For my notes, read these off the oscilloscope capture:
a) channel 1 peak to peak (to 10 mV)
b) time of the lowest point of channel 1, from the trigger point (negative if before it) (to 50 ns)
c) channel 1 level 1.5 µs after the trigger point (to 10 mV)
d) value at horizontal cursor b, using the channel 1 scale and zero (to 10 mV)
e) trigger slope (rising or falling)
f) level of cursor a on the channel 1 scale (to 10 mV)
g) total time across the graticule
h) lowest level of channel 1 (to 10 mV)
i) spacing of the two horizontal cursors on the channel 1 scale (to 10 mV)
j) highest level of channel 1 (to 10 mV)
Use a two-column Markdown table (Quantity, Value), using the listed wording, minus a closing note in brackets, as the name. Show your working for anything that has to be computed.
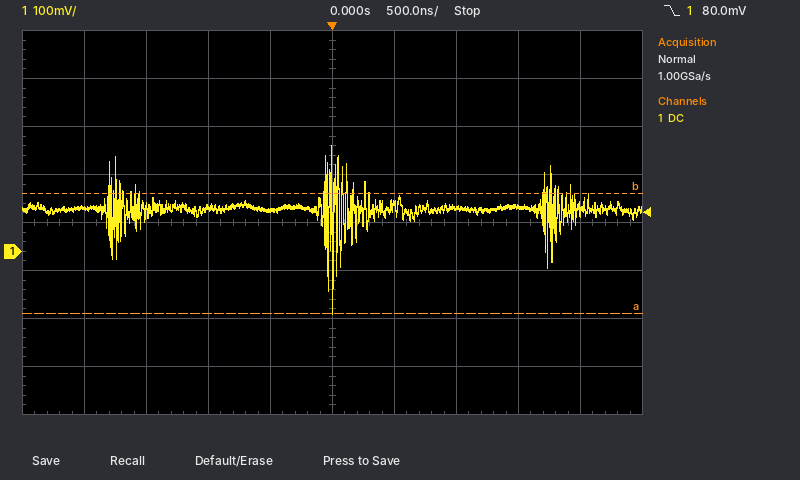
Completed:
| Quantity | Value |
|---|---|
| channel 1 peak to peak | 220 mV − (-130 mV) = 350 mV |
| time of the lowest point of channel 1, from the trigger point (negative if before it) | 0 ns |
| channel 1 level 1.5 µs after the trigger point | 90 mV |
| value at horizontal cursor b, using the channel 1 scale and zero | 120 mV |
| trigger slope | falling |
| level of cursor a on the channel 1 scale | -130 mV |
| total time across the graticule | 5 µs |
| lowest level of channel 1 | -130 mV |
| spacing of the two horizontal cursors on the channel 1 scale | 250 mV |
| highest level of channel 1 | 220 mV |
